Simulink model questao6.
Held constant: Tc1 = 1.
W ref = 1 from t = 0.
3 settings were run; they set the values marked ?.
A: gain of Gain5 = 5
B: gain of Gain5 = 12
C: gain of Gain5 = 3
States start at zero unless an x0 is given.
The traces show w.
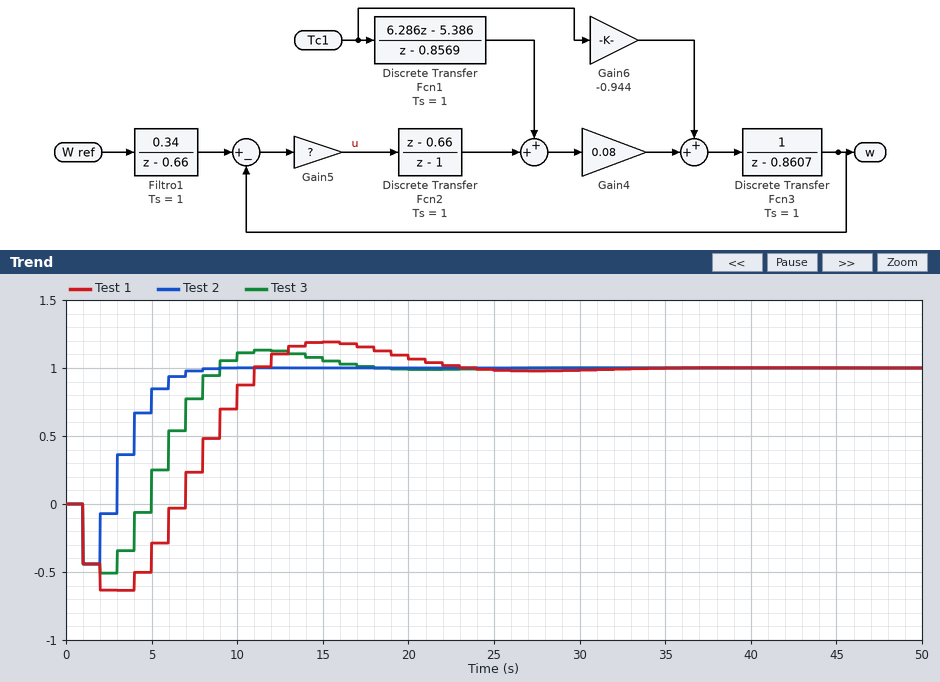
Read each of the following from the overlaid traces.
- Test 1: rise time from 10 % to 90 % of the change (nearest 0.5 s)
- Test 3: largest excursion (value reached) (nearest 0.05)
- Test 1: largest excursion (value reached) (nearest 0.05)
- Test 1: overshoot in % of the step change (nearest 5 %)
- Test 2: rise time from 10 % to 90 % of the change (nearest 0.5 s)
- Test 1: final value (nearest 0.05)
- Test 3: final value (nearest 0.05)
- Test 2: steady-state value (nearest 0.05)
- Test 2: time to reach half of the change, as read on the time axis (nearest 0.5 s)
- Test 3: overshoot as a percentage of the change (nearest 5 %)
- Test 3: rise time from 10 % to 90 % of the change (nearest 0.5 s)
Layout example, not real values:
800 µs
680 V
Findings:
4.0 s
1.15
1.20
20 %
3.0 s
1.00
1.00
1.00
4.0 s
15 %
3.0 s
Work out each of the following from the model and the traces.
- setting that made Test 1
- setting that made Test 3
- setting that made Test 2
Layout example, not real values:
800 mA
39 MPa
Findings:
C
A
B
